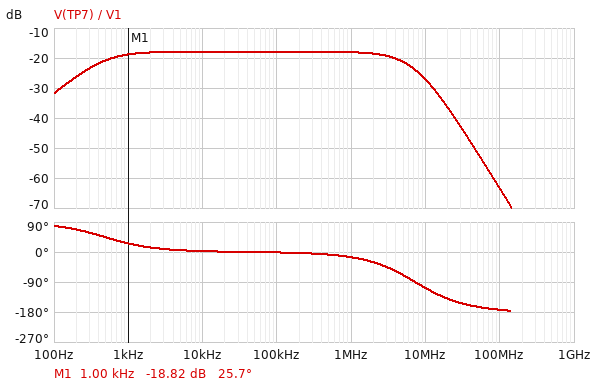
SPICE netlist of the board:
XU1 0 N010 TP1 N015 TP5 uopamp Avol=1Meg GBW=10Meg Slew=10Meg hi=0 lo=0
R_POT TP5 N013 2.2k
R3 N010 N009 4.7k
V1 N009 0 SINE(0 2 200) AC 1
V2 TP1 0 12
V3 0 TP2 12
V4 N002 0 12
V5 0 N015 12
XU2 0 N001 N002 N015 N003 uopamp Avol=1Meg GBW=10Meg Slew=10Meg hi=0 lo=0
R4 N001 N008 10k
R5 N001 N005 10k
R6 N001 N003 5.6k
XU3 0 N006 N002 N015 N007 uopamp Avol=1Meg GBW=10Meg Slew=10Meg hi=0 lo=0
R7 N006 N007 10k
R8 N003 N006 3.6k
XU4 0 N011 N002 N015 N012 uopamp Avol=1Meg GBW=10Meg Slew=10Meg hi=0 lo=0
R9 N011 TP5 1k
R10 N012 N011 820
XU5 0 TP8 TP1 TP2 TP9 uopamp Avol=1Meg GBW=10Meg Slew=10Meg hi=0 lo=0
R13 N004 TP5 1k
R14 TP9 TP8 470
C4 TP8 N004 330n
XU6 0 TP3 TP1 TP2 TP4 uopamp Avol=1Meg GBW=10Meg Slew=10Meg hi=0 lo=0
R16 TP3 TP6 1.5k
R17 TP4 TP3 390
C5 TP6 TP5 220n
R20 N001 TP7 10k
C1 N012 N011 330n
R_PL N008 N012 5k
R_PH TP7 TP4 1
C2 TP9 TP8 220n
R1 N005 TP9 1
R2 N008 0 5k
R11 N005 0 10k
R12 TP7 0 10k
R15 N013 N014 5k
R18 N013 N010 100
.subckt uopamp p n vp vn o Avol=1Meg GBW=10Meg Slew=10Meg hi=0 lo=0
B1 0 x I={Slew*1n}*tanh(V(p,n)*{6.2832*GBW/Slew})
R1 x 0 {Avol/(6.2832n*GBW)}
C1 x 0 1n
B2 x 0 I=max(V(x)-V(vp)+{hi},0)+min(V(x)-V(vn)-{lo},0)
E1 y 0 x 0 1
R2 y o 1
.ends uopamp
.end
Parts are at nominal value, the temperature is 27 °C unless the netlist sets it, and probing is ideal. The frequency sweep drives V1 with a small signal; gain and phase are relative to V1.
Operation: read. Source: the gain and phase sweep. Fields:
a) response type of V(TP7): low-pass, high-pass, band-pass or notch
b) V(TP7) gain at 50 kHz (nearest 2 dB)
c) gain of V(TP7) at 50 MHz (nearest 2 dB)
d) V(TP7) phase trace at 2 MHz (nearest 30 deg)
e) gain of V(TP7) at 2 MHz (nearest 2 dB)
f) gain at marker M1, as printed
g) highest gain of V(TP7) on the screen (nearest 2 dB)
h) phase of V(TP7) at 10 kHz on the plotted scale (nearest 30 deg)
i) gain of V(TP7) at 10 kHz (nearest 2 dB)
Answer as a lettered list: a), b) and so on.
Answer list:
a) band-pass
b) -18 dB
c) -52 dB
d) -30 deg
e) -18 dB
f) -18.82 dB
g) -18 dB
h) 0 deg
i) -18 dB
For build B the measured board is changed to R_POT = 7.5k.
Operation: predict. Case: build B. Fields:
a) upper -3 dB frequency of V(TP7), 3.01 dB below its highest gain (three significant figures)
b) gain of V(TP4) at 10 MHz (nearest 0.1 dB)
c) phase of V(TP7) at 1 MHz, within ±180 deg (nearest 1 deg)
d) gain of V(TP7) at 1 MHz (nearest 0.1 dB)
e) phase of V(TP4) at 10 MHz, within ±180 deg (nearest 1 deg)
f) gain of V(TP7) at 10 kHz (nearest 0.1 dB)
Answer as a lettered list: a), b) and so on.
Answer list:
a) 3.23 MHz
b) -20.6 dB
c) -22 deg
d) -7.9 dB
e) -121 deg
f) -7.5 dB
